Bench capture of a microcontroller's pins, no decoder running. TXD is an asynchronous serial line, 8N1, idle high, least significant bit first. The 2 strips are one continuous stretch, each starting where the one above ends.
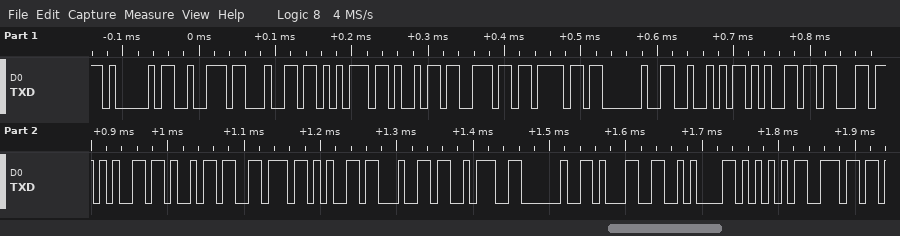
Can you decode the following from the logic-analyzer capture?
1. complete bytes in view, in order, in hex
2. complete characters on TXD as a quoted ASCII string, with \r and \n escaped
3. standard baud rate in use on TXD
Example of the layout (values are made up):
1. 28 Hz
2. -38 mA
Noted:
1. 41 72 64 75 69 6E 6F 20 52 65 63 65 69 76 65 64 3A 20 31 0A 55 6E
2. "Arduino Received: 1\nUn"
3. 115200 baud
